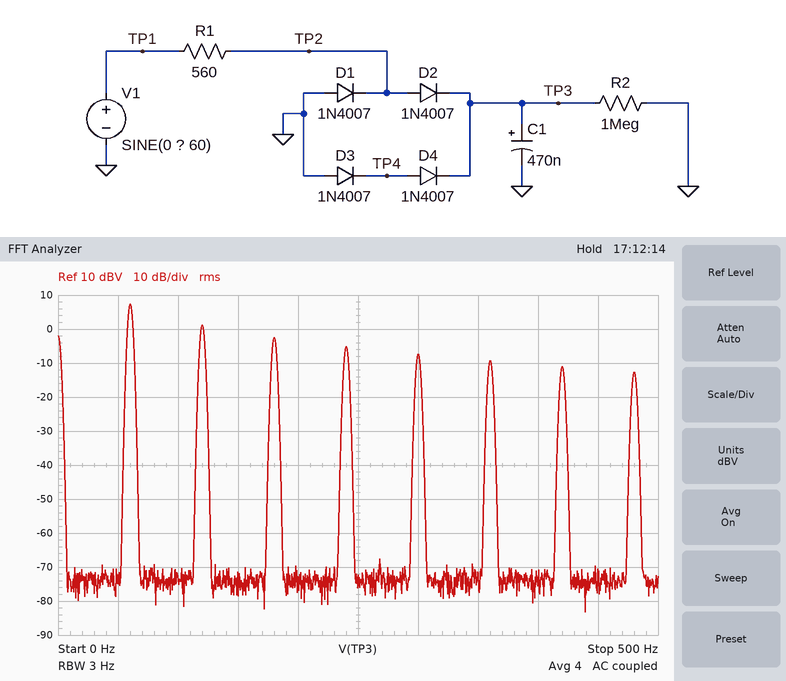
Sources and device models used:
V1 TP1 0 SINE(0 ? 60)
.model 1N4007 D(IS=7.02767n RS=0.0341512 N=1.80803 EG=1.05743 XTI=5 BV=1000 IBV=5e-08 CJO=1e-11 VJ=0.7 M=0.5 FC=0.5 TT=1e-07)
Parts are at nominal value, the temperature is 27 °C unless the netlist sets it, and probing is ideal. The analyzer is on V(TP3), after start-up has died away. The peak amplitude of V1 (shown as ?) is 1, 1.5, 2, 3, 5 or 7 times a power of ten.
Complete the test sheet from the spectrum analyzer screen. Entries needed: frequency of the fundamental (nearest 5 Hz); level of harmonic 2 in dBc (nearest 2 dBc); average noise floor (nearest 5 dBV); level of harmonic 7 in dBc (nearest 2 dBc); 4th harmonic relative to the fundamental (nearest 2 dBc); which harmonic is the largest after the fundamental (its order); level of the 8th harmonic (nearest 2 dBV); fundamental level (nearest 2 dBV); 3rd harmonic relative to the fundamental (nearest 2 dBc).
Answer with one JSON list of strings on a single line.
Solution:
["60 Hz", "-6 dBc", "-75 dBV", "-18 dBc", "-12 dBc", "2", "-12 dBV", "8 dBV", "-10 dBc"]
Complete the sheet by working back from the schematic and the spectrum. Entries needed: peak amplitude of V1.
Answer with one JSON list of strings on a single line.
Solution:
["300 V"]
